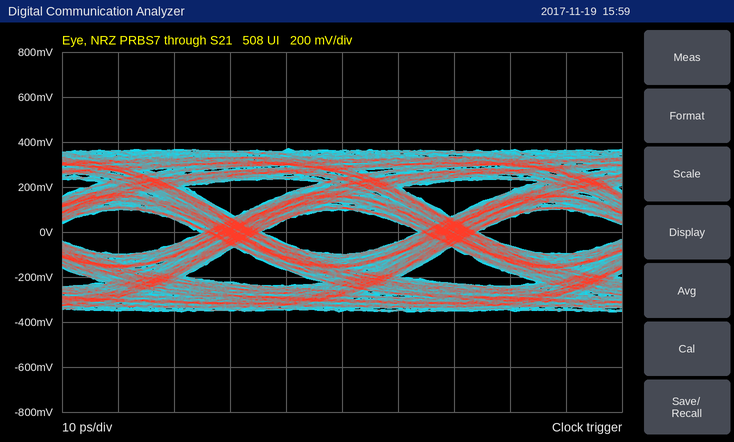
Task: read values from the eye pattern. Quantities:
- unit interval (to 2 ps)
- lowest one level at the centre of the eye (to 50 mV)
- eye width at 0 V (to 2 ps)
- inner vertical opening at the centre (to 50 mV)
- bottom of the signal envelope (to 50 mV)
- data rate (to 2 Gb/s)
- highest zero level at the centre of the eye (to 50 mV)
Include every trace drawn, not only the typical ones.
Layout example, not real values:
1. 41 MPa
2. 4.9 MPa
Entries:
1. 38 ps
2. 100 mV
3. 28 ps
4. 200 mV
5. -350 mV
6. 26 Gb/s
7. -100 mV
